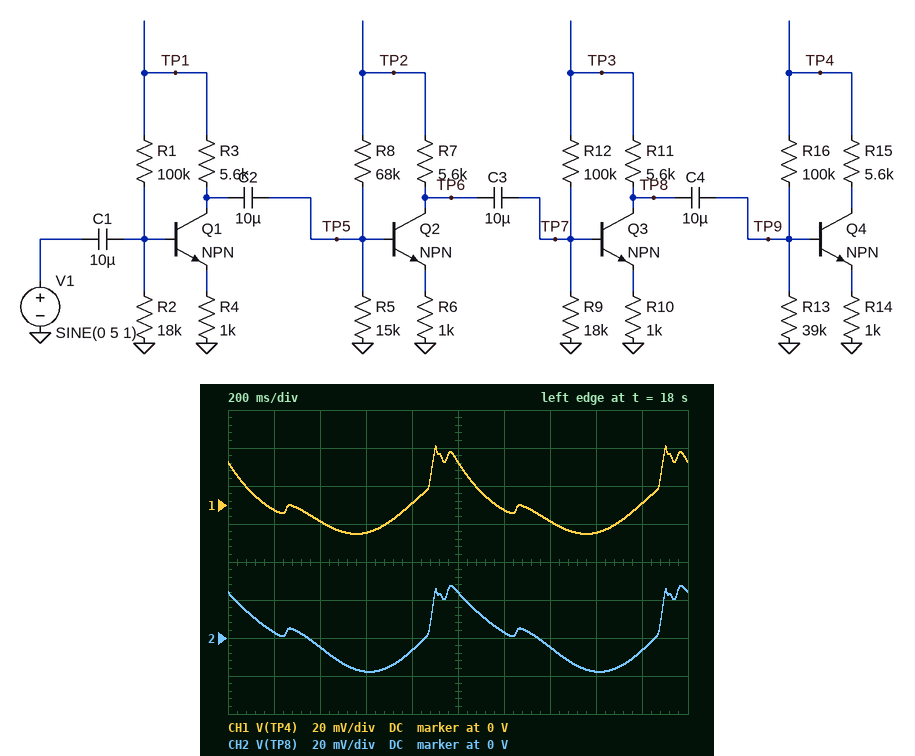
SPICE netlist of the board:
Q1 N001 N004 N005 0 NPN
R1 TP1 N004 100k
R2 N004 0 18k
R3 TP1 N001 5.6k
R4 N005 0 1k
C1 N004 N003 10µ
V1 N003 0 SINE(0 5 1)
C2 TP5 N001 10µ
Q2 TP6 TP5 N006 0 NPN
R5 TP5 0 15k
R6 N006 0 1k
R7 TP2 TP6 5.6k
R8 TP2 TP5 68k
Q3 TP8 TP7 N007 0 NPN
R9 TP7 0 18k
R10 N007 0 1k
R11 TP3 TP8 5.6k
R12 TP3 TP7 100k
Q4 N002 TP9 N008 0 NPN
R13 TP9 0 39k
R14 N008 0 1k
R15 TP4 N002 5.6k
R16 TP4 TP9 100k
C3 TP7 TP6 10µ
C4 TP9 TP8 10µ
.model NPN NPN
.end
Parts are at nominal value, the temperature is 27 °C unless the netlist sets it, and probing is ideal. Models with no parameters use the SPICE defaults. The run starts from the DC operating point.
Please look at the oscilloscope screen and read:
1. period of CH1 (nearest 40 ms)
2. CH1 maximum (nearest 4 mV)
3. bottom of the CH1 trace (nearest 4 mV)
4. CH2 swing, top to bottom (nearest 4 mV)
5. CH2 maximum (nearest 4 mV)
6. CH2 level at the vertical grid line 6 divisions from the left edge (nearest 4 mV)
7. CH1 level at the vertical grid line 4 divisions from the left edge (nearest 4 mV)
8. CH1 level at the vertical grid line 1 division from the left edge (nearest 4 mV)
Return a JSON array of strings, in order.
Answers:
["1.00 s", "32 mV", "-16 mV", "44 mV", "28 mV", "4 mV", "0 V", "-4 mV"]
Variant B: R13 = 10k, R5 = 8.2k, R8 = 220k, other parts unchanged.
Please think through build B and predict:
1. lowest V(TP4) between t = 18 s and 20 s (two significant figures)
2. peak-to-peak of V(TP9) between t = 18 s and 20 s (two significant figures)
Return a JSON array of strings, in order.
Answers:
["-1.2 mV", "4.5 mV"]
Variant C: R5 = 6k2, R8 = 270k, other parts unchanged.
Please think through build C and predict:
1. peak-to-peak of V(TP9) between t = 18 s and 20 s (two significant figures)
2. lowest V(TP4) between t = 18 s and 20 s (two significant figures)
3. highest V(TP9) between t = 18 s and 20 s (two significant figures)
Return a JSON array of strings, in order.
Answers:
["11 mV", "-2.5 mV", "8.4 mV"]
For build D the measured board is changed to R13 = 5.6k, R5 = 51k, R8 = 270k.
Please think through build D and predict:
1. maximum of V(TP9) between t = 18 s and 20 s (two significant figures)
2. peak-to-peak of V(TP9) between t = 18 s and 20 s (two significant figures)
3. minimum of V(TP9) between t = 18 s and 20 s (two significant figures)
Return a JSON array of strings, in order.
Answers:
["6.9 mV", "9.3 mV", "-2.4 mV"]
